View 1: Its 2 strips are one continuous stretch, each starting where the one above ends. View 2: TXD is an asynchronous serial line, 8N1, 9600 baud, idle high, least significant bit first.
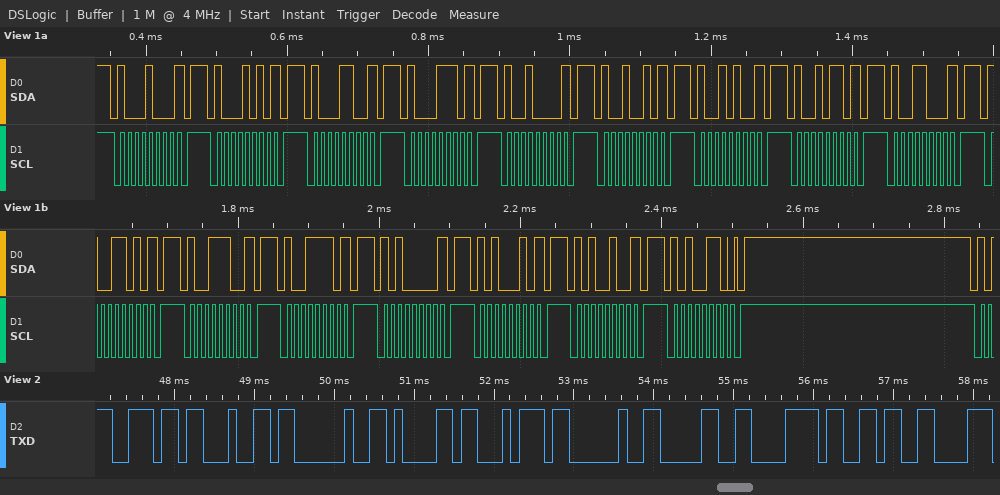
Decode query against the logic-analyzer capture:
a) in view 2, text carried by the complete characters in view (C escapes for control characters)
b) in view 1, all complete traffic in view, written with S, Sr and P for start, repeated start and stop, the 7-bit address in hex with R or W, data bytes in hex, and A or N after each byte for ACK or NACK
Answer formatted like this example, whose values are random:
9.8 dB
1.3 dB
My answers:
"nd at 0x6"
S 44W N P S 45W N P S 46W N P S 47W N P S 48W N P S 49W N P S 4AW N P S 4BW N P S 4CW N P S 4DW N P S 4EW N P S 4FW N P S 50W N P S 51W N P S 52W N P S 53W A P
